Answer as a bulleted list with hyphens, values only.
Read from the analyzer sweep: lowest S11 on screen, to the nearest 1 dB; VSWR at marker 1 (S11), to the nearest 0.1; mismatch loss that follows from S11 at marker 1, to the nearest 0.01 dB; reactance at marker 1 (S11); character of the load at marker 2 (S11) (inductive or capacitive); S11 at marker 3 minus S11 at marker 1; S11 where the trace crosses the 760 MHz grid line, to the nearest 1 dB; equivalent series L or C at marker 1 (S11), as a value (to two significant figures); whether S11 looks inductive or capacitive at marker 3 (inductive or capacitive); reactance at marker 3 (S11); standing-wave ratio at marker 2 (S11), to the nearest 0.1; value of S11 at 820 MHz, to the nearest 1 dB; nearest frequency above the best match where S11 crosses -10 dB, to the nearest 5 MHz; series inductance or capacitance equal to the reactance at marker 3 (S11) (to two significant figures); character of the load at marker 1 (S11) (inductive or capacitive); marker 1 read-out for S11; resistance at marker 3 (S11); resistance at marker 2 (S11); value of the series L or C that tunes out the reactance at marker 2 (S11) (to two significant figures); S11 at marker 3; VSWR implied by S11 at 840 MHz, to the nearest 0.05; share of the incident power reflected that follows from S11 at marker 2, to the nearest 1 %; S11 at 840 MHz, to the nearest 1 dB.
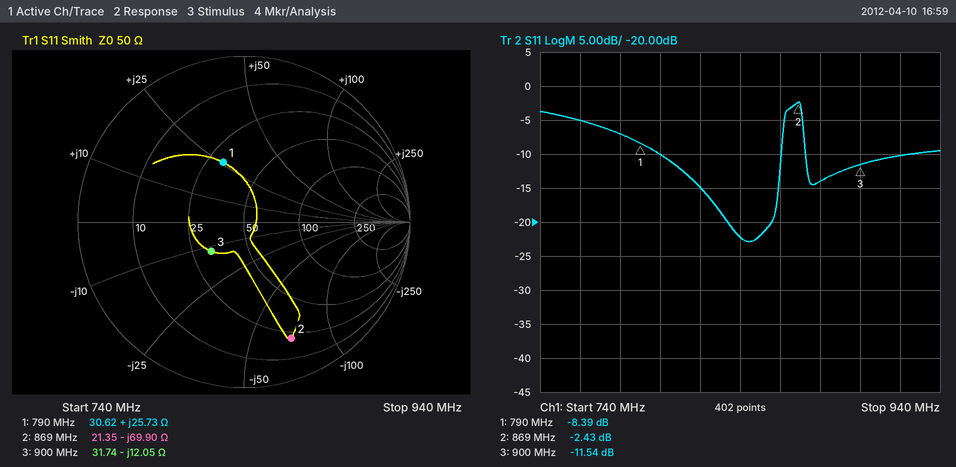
- -23 dB
- 2.2
- 0.68 dB
- +25.73 Ω
- capacitive
- -3.15 dB
- -5 dB
- 5.2 nH
- capacitive
- -12.05 Ω
- 7.2
- -15 dB
- 860 MHz
- 15 pF
- inductive
- -8.39 dB
- 31.74 Ω
- 21.35 Ω
- 13 nH
- -11.54 dB
- 1.15
- 57 %
- -22 dB
